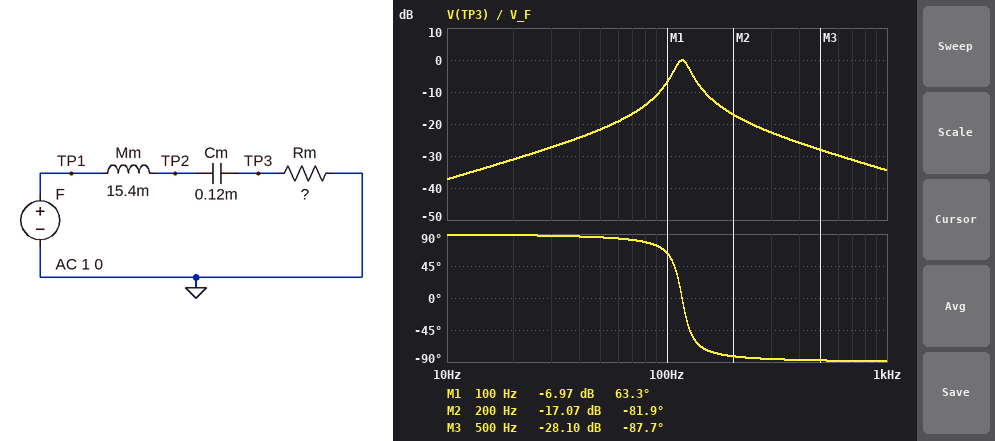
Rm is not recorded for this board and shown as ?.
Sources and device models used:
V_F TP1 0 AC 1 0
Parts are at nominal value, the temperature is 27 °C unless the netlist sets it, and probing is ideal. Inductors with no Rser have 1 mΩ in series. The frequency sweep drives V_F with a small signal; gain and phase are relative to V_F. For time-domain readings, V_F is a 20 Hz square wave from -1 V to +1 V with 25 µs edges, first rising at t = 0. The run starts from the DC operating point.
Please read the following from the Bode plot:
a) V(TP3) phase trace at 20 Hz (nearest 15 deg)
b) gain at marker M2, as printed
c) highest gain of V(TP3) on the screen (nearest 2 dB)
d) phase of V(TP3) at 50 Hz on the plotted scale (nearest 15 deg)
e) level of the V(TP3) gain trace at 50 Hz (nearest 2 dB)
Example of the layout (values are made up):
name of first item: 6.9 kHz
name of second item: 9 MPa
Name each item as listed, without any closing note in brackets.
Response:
V(TP3) phase trace at 20 Hz: 90 deg
gain at marker M2, as printed: -17.07 dB
highest gain of V(TP3) on the screen: 0 dB
phase of V(TP3) at 50 Hz on the plotted scale: 90 deg
level of the V(TP3) gain trace at 50 Hz: -22 dB
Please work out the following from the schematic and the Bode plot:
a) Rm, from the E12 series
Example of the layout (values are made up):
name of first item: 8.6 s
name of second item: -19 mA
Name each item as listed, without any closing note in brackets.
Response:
Rm, from the E12 series: 1.8 Ω
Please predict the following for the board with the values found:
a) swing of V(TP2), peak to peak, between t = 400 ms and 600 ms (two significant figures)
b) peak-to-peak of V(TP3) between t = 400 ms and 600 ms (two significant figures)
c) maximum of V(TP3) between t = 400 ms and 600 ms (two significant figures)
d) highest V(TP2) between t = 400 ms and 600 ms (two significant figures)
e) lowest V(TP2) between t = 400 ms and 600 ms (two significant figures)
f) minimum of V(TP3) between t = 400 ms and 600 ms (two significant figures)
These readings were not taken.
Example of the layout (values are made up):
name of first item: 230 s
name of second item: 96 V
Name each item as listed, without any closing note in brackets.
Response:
swing of V(TP2), peak to peak, between t = 400 ms and 600 ms: 4.6 V
peak-to-peak of V(TP3) between t = 400 ms and 600 ms: 470 mV
maximum of V(TP3) between t = 400 ms and 600 ms: 240 mV
highest V(TP2) between t = 400 ms and 600 ms: 2.3 V
lowest V(TP2) between t = 400 ms and 600 ms: -2.3 V
minimum of V(TP3) between t = 400 ms and 600 ms: -240 mV
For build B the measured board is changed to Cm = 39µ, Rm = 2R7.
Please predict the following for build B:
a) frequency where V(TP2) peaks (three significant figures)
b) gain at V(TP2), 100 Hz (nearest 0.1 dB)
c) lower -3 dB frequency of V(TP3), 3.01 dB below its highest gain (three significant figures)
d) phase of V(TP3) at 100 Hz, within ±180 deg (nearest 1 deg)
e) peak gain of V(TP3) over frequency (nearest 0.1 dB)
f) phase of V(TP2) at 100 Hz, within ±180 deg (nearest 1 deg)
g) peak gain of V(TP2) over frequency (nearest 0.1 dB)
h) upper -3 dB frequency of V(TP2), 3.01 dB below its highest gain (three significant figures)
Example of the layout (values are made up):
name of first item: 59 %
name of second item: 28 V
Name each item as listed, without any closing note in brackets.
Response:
frequency where V(TP2) peaks: 204 Hz
gain at V(TP2), 100 Hz: 2.3 dB
lower -3 dB frequency of V(TP3), 3.01 dB below its highest gain: 192 Hz
phase of V(TP3) at 100 Hz, within ±180 deg: 85 deg
peak gain of V(TP3) over frequency: 0 dB
phase of V(TP2) at 100 Hz, within ±180 deg: -1 deg
peak gain of V(TP2) over frequency: 17.4 dB
upper -3 dB frequency of V(TP2), 3.01 dB below its highest gain: 218 Hz
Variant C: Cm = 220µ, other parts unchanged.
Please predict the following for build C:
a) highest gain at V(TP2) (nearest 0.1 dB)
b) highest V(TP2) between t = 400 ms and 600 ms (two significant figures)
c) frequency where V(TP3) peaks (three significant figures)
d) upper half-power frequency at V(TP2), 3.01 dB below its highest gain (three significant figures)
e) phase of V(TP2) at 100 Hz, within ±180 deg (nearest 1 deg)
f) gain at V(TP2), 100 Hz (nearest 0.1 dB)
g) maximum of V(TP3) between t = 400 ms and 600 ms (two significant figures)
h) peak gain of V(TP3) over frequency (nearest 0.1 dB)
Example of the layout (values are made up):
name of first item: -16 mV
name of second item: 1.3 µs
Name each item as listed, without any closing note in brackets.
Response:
highest gain at V(TP2): 13.6 dB
highest V(TP2) between t = 400 ms and 600 ms: 2.2 V
frequency where V(TP3) peaks: 86.5 Hz
upper half-power frequency at V(TP2), 3.01 dB below its highest gain: 94.4 Hz
phase of V(TP2) at 100 Hz, within ±180 deg: -130 deg
gain at V(TP2), 100 Hz: 7.8 dB
maximum of V(TP3) between t = 400 ms and 600 ms: 310 mV
peak gain of V(TP3) over frequency: 0 dB
